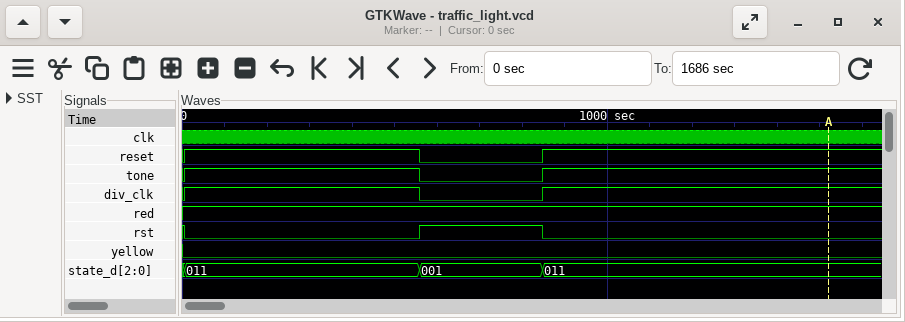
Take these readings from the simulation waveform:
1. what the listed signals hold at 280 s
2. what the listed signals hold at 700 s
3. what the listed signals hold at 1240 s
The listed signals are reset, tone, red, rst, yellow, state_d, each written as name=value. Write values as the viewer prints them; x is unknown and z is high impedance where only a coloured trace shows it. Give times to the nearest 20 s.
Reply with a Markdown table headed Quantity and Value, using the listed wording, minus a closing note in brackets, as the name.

| Quantity | Value |
|---|---|
| what the listed signals hold at 280 s | reset=1, tone=1, red=1, rst=0, yellow=0, state_d=011 |
| what the listed signals hold at 700 s | reset=0, tone=0, red=1, rst=1, yellow=0, state_d=001 |
| what the listed signals hold at 1240 s | reset=1, tone=1, red=1, rst=0, yellow=0, state_d=011 |
